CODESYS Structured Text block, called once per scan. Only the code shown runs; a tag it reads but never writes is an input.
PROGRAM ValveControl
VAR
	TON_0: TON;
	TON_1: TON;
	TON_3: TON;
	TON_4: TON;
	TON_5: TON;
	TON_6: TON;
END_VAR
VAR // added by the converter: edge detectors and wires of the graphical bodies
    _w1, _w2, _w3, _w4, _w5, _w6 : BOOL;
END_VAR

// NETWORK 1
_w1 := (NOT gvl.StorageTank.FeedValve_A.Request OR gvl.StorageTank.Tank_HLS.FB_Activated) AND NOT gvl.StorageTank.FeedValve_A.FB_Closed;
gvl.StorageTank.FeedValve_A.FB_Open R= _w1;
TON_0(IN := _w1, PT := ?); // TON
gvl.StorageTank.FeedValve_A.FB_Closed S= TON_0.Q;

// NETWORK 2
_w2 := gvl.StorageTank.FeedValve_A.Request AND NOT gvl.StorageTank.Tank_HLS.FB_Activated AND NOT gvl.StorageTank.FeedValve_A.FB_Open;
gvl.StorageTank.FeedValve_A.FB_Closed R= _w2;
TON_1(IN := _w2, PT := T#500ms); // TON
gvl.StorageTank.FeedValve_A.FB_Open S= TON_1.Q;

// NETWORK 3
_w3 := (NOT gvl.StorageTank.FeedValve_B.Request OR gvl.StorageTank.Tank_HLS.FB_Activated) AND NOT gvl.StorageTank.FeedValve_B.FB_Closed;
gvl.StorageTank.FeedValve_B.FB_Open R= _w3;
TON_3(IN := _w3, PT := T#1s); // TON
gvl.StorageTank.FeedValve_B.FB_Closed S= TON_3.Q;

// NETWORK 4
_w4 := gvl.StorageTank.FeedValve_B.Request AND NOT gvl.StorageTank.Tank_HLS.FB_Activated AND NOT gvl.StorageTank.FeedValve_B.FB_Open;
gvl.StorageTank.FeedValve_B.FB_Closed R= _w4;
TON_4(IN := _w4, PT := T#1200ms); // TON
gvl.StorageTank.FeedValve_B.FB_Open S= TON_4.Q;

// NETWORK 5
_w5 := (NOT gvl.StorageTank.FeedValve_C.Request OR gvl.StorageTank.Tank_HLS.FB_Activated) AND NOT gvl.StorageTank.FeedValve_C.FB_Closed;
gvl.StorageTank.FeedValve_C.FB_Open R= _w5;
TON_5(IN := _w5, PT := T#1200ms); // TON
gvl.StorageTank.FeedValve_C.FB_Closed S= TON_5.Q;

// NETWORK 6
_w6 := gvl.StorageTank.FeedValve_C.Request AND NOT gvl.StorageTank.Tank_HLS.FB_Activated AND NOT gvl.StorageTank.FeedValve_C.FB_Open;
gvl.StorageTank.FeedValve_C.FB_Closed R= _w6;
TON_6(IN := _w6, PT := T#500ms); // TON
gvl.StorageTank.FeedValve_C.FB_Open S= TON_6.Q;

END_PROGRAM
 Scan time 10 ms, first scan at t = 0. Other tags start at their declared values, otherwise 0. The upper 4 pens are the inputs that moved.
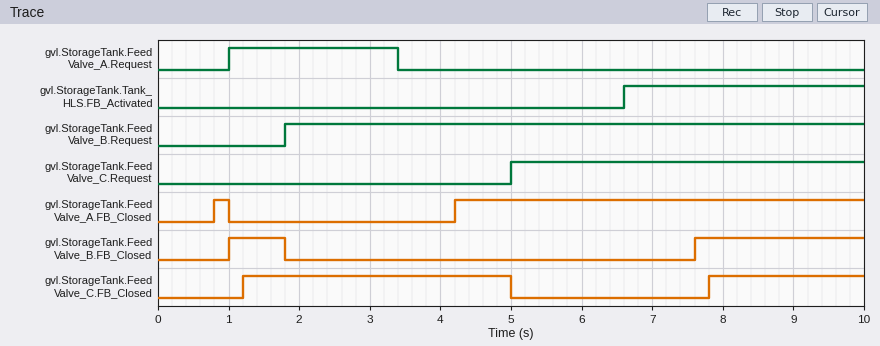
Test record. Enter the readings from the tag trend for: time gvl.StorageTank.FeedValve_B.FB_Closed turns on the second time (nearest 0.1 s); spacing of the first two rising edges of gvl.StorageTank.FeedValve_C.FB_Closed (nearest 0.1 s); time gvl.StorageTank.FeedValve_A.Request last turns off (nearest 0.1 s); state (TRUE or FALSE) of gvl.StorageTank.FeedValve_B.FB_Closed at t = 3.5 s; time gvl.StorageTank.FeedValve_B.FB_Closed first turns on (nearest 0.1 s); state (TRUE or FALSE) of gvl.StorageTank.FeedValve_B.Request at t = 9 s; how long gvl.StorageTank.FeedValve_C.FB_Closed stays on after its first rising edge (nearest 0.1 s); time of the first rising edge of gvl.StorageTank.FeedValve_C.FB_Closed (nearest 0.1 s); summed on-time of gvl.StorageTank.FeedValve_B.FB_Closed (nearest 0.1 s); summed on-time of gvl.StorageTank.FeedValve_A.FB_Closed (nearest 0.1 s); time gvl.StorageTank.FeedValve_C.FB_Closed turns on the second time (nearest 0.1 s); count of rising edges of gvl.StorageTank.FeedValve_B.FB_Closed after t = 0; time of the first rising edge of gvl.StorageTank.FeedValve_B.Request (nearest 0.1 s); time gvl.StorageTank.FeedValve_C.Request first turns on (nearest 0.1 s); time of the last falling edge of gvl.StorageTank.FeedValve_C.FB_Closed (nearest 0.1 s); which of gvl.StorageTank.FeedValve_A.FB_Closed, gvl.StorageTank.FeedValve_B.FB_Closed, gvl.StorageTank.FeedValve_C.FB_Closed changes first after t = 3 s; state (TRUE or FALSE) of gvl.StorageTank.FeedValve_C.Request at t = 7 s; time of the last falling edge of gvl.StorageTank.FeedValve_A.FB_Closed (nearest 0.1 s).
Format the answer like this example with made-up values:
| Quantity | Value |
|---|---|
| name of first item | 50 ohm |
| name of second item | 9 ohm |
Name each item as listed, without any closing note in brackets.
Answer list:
| Quantity | Value |
|---|---|
| time gvl.StorageTank.FeedValve_B.FB_Closed turns on the second time | 7.6 s |
| spacing of the first two rising edges of gvl.StorageTank.FeedValve_C.FB_Closed | 6.6 s |
| time gvl.StorageTank.FeedValve_A.Request last turns off | 3.4 s |
| state (TRUE or FALSE) of gvl.StorageTank.FeedValve_B.FB_Closed at t = 3.5 s | FALSE |
| time gvl.StorageTank.FeedValve_B.FB_Closed first turns on | 1.0 s |
| state (TRUE or FALSE) of gvl.StorageTank.FeedValve_B.Request at t = 9 s | TRUE |
| how long gvl.StorageTank.FeedValve_C.FB_Closed stays on after its first rising edge | 3.8 s |
| time of the first rising edge of gvl.StorageTank.FeedValve_C.FB_Closed | 1.2 s |
| summed on-time of gvl.StorageTank.FeedValve_B.FB_Closed | 3.2 s |
| summed on-time of gvl.StorageTank.FeedValve_A.FB_Closed | 6.0 s |
| time gvl.StorageTank.FeedValve_C.FB_Closed turns on the second time | 7.8 s |
| count of rising edges of gvl.StorageTank.FeedValve_B.FB_Closed after t = 0 | 2 |
| time of the first rising edge of gvl.StorageTank.FeedValve_B.Request | 1.8 s |
| time gvl.StorageTank.FeedValve_C.Request first turns on | 5.0 s |
| time of the last falling edge of gvl.StorageTank.FeedValve_C.FB_Closed | 5.0 s |
| which of gvl.StorageTank.FeedValve_A.FB_Closed, gvl.StorageTank.FeedValve_B.FB_Closed, gvl.StorageTank.FeedValve_C.FB_Closed changes first after t = 3 s | gvl.StorageTank.FeedValve_A.FB_Closed |
| state (TRUE or FALSE) of gvl.StorageTank.FeedValve_C.Request at t = 7 s | TRUE |
| time of the last falling edge of gvl.StorageTank.FeedValve_A.FB_Closed | 1.0 s |
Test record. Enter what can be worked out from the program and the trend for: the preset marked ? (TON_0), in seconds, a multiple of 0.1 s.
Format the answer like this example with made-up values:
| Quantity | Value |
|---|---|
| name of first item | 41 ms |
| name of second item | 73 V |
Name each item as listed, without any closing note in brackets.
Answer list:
| Quantity | Value |
|---|---|
| the preset marked ? (TON_0), in seconds, a multiple of 0.1 s | 0.8 s |
